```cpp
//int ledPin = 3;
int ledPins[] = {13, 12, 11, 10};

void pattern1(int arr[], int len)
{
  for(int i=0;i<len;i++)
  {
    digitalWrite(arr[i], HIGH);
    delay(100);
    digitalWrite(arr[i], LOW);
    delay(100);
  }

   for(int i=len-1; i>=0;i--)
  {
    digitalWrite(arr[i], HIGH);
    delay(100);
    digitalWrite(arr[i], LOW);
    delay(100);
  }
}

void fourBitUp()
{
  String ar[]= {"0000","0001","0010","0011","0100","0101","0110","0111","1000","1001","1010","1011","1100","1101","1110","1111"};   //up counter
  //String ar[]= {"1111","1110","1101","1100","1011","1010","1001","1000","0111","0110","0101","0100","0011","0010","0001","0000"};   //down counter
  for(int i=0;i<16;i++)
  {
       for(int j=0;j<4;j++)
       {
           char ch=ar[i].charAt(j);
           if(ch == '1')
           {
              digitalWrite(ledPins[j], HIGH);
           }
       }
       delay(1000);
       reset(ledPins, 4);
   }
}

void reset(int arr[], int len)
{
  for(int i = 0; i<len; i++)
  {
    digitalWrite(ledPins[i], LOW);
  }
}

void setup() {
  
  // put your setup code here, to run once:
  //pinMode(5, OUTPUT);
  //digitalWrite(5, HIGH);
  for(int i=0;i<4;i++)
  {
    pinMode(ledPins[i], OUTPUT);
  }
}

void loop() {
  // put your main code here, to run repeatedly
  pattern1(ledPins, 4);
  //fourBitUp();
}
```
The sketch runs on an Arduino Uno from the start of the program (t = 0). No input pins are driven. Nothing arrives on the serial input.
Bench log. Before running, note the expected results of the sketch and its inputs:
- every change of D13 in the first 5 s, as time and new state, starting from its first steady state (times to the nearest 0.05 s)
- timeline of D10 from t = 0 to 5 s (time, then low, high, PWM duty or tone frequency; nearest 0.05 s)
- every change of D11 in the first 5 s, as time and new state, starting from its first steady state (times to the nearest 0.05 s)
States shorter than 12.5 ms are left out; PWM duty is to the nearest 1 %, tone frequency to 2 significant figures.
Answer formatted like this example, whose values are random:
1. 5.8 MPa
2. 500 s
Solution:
1. 0 s high; 0.1 s low; 1.4 s high; 1.5 s low; 1.6 s high; 1.7 s low; 3 s high; 3.1 s low; 3.2 s high; 3.3 s low; 4.6 s high; 4.7 s low; 4.8 s high; 4.9 s low
2. 0 s low; 0.6 s high; 0.7 s low; 0.8 s high; 0.9 s low; 2.2 s high; 2.3 s low; 2.4 s high; 2.5 s low; 3.8 s high; 3.9 s low; 4 s high; 4.1 s low
3. 0 s low; 0.4 s high; 0.5 s low; 1 s high; 1.1 s low; 2 s high; 2.1 s low; 2.6 s high; 2.7 s low; 3.6 s high; 3.7 s low; 4.2 s high; 4.3 s low
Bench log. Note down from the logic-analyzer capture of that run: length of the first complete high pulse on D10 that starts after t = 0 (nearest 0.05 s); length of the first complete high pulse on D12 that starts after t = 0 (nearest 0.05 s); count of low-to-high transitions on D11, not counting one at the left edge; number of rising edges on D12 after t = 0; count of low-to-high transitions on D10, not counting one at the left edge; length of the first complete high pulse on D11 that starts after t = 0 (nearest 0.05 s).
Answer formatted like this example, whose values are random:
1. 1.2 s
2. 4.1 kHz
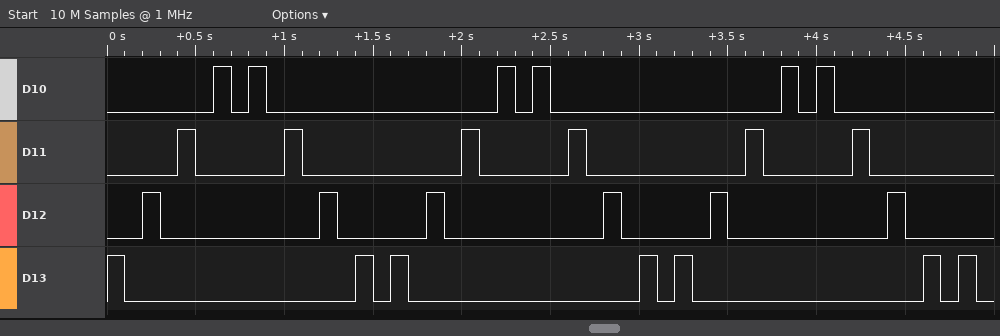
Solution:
1. 0.10 s
2. 0.10 s
3. 6
4. 6
5. 6
6. 0.10 s
